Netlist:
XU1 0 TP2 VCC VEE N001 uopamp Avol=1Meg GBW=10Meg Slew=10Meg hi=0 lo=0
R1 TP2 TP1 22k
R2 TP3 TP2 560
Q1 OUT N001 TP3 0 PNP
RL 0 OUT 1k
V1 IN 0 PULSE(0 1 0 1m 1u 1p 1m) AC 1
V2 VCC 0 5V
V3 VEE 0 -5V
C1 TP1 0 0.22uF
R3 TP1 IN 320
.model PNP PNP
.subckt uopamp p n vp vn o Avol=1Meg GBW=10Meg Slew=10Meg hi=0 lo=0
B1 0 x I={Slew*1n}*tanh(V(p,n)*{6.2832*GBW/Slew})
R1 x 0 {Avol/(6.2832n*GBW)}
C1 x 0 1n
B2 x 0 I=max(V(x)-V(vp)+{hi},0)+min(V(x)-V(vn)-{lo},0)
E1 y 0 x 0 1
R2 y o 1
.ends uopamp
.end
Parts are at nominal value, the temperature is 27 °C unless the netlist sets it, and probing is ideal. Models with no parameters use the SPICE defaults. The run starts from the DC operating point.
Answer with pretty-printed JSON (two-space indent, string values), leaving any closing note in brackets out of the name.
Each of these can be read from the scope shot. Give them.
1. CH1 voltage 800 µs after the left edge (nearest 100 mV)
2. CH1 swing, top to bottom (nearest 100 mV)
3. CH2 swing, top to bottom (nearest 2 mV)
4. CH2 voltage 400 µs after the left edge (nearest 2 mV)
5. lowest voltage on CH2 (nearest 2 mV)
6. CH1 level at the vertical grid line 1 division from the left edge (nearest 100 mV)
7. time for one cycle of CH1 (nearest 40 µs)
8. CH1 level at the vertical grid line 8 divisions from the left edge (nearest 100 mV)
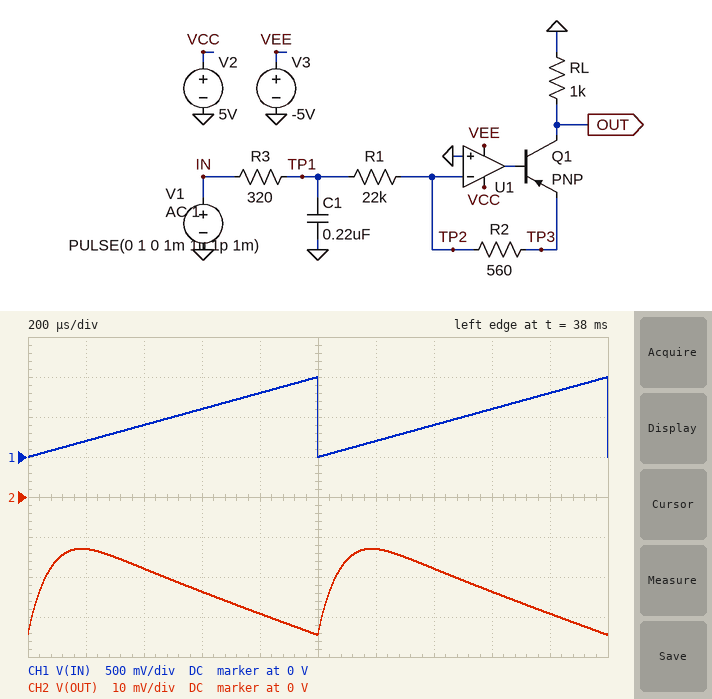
{
  "CH1 voltage 800 µs after the left edge": "800 mV",
  "CH1 swing, top to bottom": "1.0 V",
  "CH2 swing, top to bottom": "22 mV",
  "CH2 voltage 400 µs after the left edge": "-18 mV",
  "lowest voltage on CH2": "-34 mV",
  "CH1 level at the vertical grid line 1 division from the left edge": "200 mV",
  "time for one cycle of CH1": "1.00 ms",
  "CH1 level at the vertical grid line 8 divisions from the left edge": "600 mV"
}
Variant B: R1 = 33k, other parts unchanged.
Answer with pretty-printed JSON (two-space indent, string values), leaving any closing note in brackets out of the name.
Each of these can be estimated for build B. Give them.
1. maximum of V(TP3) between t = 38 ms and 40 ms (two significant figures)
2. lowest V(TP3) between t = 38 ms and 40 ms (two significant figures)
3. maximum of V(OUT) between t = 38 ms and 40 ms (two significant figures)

{
  "maximum of V(TP3) between t = 38 ms and 40 ms": "-3.1 mV",
  "lowest V(TP3) between t = 38 ms and 40 ms": "-16 mV",
  "maximum of V(OUT) between t = 38 ms and 40 ms": "-11 mV"
}
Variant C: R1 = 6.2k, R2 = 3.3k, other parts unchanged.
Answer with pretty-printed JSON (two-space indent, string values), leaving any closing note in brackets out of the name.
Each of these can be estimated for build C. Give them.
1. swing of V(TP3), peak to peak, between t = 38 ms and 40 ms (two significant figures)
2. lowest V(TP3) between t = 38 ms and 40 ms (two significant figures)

{
  "swing of V(TP3), peak to peak, between t = 38 ms and 40 ms": "380 mV",
  "lowest V(TP3) between t = 38 ms and 40 ms": "-470 mV"
}
